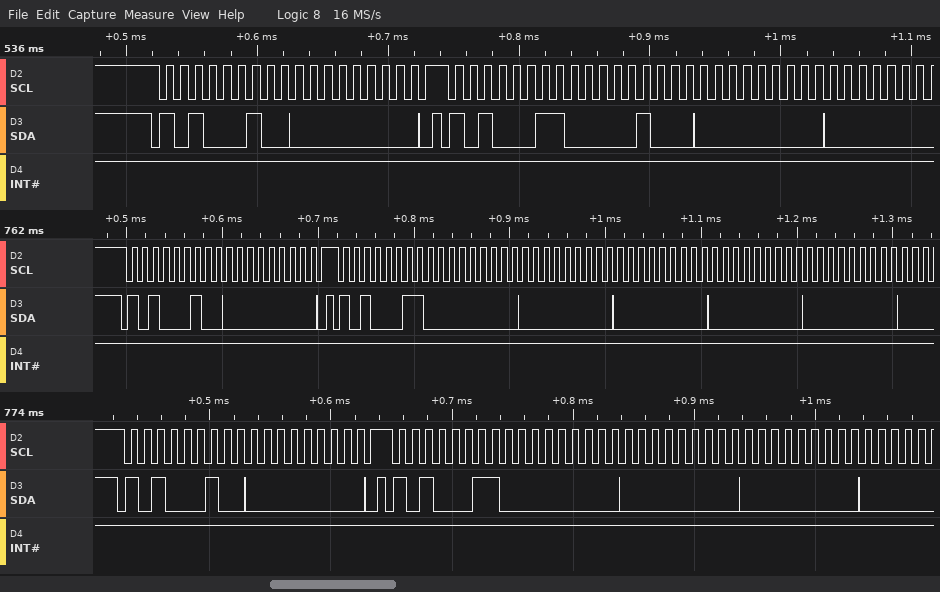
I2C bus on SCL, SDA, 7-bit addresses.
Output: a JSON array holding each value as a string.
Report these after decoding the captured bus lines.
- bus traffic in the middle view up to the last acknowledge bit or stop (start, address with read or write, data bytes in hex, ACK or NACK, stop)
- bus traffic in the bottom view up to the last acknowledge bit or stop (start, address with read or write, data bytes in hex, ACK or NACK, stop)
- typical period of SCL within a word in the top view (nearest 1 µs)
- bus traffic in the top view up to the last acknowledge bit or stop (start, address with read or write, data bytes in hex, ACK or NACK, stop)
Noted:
["start, address 51 write ACK, 00 ACK, stop, start, address 51 read ACK, 00 ACK, 00 ACK, 00 ACK, 00 ACK, 00 ACK", "start, address 51 write ACK, 00 ACK, stop, start, address 51 read ACK, 00 ACK, 00 ACK, 00 ACK", "11 µs", "start, address 51 write ACK, 00 ACK, stop, start, address 51 read ACK, 08 ACK, 00 ACK"]
